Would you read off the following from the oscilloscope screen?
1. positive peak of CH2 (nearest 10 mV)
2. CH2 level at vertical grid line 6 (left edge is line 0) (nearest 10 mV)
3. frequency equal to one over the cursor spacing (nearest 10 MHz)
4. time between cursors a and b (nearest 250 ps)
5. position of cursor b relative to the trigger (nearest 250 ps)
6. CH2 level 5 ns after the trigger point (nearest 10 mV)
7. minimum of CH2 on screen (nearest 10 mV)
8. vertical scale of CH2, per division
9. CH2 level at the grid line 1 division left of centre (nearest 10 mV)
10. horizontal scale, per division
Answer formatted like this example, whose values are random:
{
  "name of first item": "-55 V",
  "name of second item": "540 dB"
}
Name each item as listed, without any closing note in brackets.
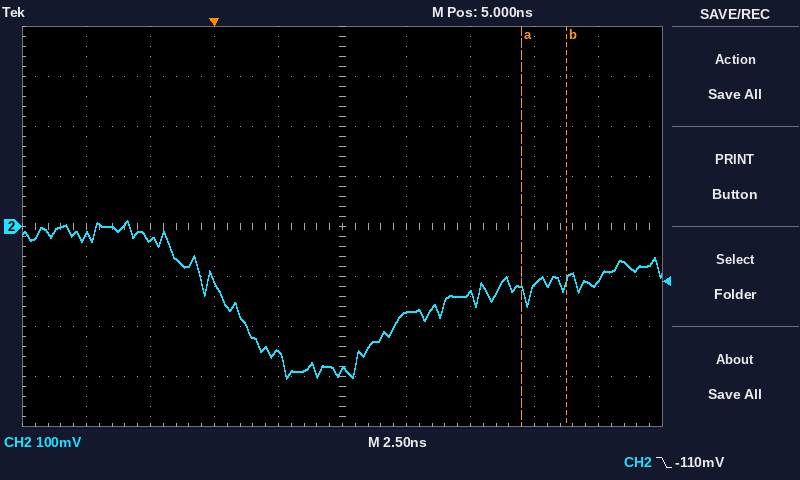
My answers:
{
  "positive peak of CH2": "10 mV",
  "CH2 level at vertical grid line 6 (left edge is line 0)": "-170 mV",
  "frequency equal to one over the cursor spacing": "570 MHz",
  "time between cursors a and b": "1.75 ns",
  "position of cursor b relative to the trigger": "+13.75 ns",
  "CH2 level 5 ns after the trigger point": "-290 mV",
  "minimum of CH2 on screen": "-300 mV",
  "vertical scale of CH2, per division": "100 mV",
  "CH2 level at the grid line 1 division left of centre": "-250 mV",
  "horizontal scale, per division": "2.5 ns"
}
